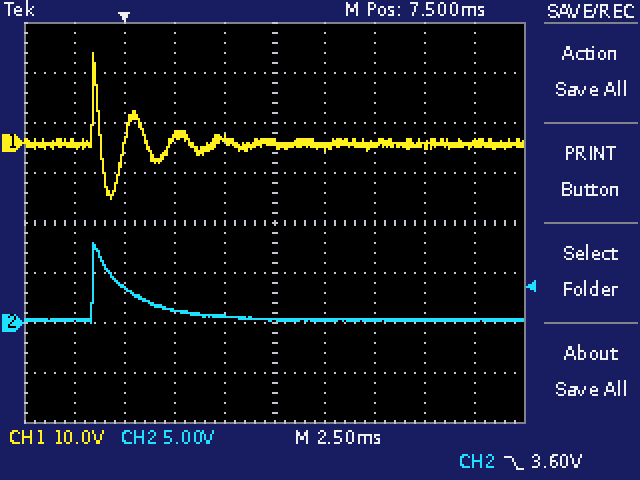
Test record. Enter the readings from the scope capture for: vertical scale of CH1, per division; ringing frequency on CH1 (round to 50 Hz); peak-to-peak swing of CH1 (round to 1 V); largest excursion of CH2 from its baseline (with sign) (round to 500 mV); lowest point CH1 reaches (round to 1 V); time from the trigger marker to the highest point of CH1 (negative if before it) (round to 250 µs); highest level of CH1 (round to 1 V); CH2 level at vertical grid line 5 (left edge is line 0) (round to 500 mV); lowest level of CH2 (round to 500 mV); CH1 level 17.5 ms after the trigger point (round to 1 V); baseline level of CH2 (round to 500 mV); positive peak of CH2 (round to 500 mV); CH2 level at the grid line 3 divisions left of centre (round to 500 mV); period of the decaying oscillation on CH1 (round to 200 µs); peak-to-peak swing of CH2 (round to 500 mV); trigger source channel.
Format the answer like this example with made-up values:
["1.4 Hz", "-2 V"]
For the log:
["10 V", "450 Hz", "29 V", "+7.5 V", "-11 V", "-1.50 ms", "18 V", "500 mV", "0.0 V", "0 V", "500 mV", "8.0 V", "3.5 V", "2.2 ms", "8.0 V", "CH2"]
